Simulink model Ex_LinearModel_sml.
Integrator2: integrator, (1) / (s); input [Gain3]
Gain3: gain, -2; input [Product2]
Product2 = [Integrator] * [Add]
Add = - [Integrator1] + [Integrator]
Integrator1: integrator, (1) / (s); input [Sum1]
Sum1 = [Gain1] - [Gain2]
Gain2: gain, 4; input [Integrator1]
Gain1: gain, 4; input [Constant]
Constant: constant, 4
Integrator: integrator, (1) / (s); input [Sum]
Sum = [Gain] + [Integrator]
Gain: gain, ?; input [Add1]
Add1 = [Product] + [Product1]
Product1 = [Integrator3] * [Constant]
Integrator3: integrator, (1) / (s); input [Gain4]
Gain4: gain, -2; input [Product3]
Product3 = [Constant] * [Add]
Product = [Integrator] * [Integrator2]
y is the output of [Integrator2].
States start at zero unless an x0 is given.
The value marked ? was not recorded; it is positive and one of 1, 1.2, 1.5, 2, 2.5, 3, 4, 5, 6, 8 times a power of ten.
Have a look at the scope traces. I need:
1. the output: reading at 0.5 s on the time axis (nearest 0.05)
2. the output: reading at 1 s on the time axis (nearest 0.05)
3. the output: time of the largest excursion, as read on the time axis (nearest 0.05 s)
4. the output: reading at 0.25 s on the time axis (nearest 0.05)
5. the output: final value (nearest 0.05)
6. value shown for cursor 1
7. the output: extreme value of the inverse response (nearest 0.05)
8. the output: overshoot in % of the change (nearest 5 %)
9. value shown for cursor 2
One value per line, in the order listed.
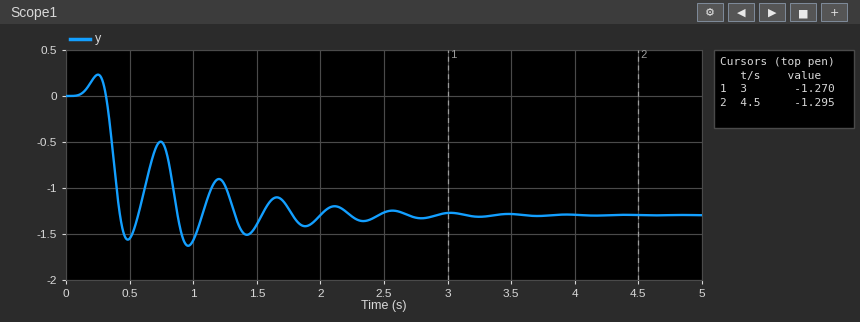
-1.55
-1.55
0.95 s
0.25
-1.30
-1.270
0.25
25 %
-1.295
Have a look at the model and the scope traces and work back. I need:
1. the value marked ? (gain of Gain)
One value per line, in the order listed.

3
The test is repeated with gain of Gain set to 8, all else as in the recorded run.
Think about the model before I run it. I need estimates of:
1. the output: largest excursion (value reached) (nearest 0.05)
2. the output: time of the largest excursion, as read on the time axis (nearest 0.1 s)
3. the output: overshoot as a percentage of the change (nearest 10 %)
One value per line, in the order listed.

-0.65
0.6 s
30 %
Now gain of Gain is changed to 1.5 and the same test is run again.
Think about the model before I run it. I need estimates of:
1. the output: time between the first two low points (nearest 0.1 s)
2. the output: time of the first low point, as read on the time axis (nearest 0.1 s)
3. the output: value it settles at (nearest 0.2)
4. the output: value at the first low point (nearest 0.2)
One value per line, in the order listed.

0.7 s
0.6 s
-2.4
-3.0
